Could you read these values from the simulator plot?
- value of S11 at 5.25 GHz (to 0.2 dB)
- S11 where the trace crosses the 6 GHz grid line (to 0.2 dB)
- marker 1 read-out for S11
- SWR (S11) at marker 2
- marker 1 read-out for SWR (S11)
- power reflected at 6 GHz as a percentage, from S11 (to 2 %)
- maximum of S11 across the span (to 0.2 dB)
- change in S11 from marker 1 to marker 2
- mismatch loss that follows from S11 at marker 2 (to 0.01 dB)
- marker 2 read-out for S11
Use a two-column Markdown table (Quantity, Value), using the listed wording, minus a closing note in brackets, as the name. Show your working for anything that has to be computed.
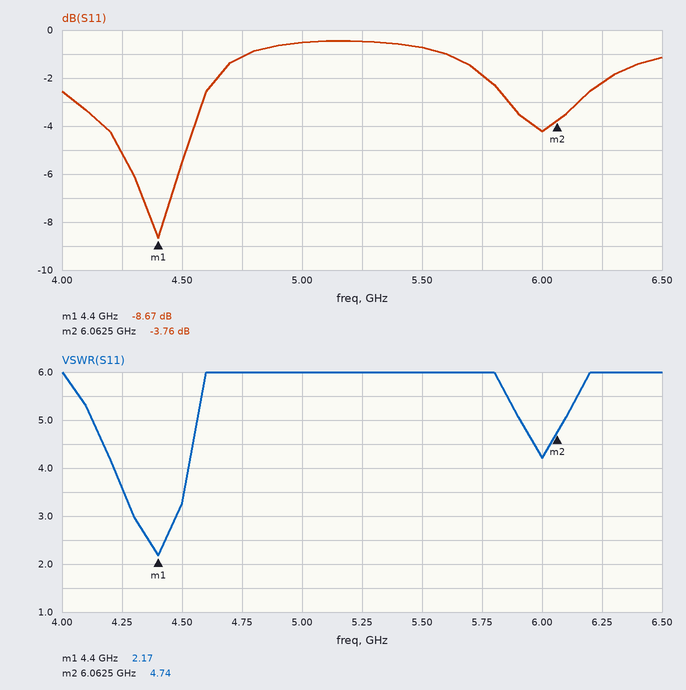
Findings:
| Quantity | Value |
|---|---|
| value of S11 at 5.25 GHz | -0.4 dB |
| S11 where the trace crosses the 6 GHz grid line | -4.2 dB |
| marker 1 read-out for S11 | -8.67 dB |
| SWR (S11) at marker 2 | 4.74 |
| marker 1 read-out for SWR | 2.17 |
| power reflected at 6 GHz as a percentage, from S11 | 10^(-4.2/10) ≈ 38 % |
| maximum of S11 across the span | -0.4 dB |
| change in S11 from marker 1 to marker 2 | -3.76 − (-8.67) = 4.91 dB |
| mismatch loss that follows from S11 at marker 2 | −10 log10(1 − 10^(-3.76/10)) ≈ 2.37 dB |
| marker 2 read-out for S11 | -3.76 dB |
